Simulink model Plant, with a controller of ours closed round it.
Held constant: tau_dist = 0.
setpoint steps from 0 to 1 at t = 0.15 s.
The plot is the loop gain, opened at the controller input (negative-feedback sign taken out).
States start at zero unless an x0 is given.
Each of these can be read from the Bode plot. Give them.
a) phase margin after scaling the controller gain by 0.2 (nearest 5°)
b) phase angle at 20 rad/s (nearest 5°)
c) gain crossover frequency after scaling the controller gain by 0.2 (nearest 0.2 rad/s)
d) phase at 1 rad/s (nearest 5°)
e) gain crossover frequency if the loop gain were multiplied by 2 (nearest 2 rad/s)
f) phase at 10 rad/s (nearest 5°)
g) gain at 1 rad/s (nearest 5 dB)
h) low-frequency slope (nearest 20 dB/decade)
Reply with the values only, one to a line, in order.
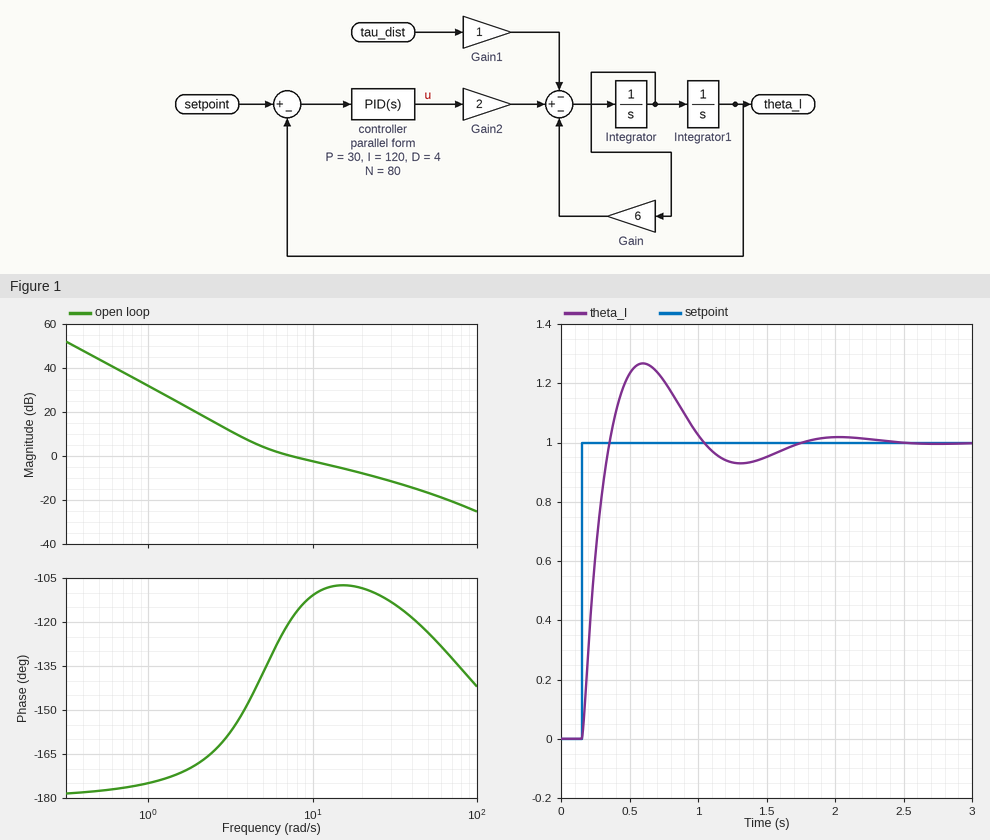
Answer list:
20°
-110°
2.8 rad/s
-175°
16 rad/s
-110°
30 dB
-40 dB/decade
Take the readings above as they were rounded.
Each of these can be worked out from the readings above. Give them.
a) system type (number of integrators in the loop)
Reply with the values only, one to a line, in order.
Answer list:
2
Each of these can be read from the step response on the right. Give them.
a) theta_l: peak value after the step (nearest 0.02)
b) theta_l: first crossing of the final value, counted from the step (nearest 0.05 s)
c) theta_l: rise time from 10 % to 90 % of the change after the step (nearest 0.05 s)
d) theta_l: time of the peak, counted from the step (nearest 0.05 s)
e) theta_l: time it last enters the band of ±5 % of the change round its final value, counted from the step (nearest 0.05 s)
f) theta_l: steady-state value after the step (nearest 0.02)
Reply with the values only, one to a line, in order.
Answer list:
1.26
0.20 s
0.15 s
0.45 s
1.35 s
1.00
